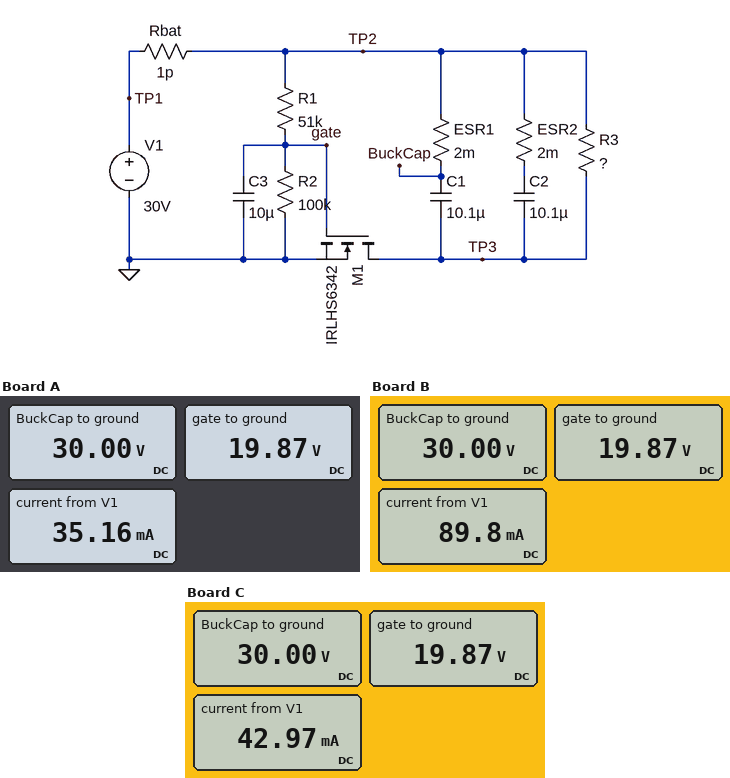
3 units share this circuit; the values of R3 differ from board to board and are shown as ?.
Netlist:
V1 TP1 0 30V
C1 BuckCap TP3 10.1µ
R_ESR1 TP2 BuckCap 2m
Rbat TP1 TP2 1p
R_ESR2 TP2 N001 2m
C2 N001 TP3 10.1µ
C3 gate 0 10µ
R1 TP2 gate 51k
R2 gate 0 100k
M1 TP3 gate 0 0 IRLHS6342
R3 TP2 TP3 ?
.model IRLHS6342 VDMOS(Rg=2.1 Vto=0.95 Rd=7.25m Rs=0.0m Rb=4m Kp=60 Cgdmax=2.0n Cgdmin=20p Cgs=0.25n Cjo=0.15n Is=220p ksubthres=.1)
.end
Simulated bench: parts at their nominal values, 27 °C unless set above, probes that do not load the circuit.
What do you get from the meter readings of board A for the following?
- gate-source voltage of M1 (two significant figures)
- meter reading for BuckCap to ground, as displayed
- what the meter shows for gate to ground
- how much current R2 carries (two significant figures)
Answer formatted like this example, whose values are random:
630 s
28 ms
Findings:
20 V
30.00 V
19.87 V
200 µA
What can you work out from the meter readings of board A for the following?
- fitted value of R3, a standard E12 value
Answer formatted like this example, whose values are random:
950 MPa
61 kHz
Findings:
820 Ω
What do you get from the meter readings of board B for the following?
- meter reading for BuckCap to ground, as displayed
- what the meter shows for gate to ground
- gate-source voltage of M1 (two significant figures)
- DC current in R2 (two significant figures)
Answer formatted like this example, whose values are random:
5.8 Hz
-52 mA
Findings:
30.00 V
19.87 V
20 V
200 µA
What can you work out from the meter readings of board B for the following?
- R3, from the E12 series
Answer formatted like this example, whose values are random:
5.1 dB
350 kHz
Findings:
330 Ω
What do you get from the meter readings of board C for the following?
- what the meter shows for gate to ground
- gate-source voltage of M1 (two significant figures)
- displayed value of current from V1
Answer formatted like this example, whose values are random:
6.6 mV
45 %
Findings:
19.87 V
20 V
42.97 mA
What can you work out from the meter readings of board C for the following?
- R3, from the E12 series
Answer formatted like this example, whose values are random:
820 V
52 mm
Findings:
680 Ω
